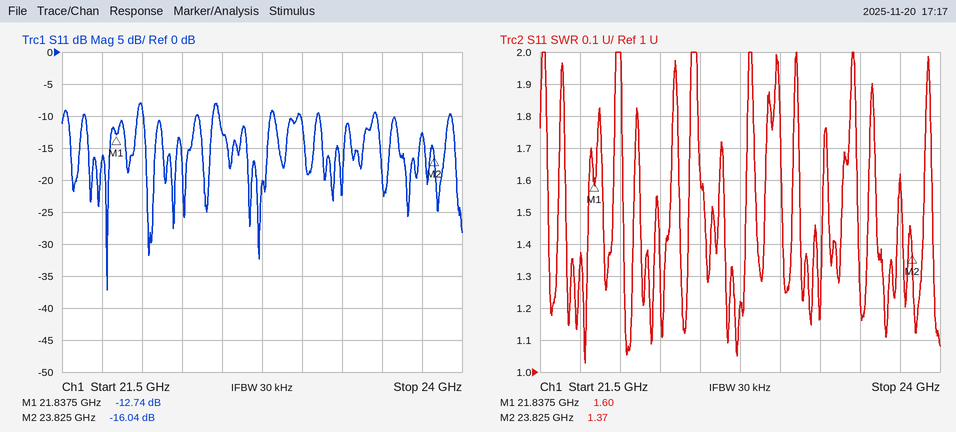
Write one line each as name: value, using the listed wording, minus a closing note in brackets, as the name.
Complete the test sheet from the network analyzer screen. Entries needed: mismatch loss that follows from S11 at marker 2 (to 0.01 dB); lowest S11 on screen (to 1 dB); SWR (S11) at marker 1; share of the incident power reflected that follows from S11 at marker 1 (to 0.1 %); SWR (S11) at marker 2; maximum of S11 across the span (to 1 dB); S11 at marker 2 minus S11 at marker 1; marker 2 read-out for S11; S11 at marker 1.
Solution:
mismatch loss that follows from S11 at marker 2: 0.11 dB
lowest S11 on screen: -37 dB
SWR (S11) at marker 1: 1.60
share of the incident power reflected that follows from S11 at marker 1: 5.3 %
SWR (S11) at marker 2: 1.37
maximum of S11 across the span: -8 dB
S11 at marker 2 minus S11 at marker 1: -3.30 dB
marker 2 read-out for S11: -16.04 dB
S11 at marker 1: -12.74 dB
